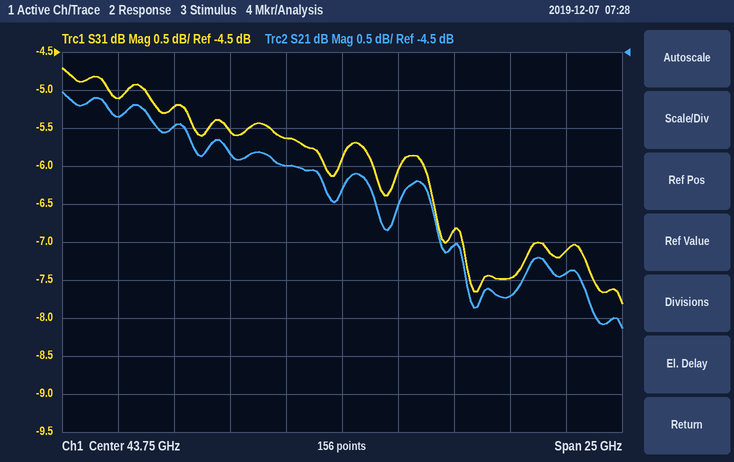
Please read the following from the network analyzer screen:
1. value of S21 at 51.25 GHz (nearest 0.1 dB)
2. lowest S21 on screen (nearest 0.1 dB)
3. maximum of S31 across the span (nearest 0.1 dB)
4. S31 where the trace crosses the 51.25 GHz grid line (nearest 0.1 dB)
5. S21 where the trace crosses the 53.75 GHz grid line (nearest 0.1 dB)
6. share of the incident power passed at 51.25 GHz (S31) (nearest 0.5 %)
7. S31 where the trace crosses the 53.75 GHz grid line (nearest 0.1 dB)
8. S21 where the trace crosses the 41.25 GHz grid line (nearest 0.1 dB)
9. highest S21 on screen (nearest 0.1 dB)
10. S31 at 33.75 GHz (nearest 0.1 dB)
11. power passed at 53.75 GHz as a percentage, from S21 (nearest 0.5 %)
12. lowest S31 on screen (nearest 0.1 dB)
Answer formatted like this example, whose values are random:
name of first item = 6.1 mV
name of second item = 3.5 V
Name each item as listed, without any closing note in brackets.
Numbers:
value of S21 at 51.25 GHz = -7.7 dB
lowest S21 on screen = -8.1 dB
maximum of S31 across the span = -4.7 dB
S31 where the trace crosses the 51.25 GHz grid line = -7.5 dB
S21 where the trace crosses the 53.75 GHz grid line = -7.4 dB
share of the incident power passed at 51.25 GHz (S31) = 18.0 %
S31 where the trace crosses the 53.75 GHz grid line = -7.1 dB
S21 where the trace crosses the 41.25 GHz grid line = -6.0 dB
highest S21 on screen = -5.0 dB
S31 at 33.75 GHz = -5.1 dB
power passed at 53.75 GHz as a percentage, from S21 = 18.0 %
lowest S31 on screen = -7.8 dB
